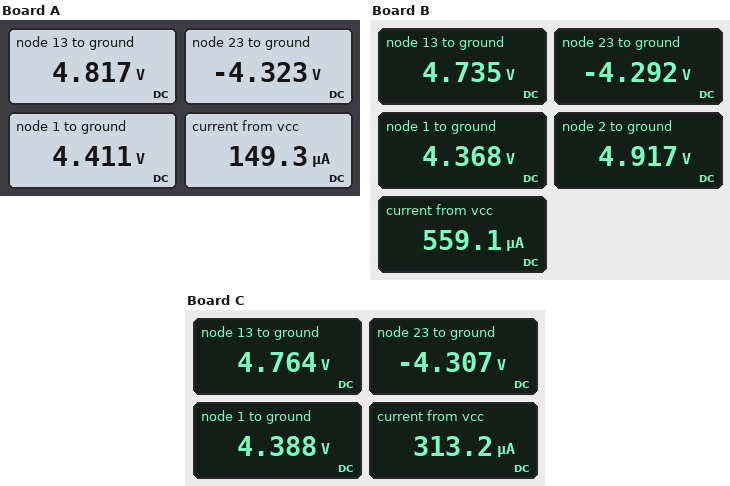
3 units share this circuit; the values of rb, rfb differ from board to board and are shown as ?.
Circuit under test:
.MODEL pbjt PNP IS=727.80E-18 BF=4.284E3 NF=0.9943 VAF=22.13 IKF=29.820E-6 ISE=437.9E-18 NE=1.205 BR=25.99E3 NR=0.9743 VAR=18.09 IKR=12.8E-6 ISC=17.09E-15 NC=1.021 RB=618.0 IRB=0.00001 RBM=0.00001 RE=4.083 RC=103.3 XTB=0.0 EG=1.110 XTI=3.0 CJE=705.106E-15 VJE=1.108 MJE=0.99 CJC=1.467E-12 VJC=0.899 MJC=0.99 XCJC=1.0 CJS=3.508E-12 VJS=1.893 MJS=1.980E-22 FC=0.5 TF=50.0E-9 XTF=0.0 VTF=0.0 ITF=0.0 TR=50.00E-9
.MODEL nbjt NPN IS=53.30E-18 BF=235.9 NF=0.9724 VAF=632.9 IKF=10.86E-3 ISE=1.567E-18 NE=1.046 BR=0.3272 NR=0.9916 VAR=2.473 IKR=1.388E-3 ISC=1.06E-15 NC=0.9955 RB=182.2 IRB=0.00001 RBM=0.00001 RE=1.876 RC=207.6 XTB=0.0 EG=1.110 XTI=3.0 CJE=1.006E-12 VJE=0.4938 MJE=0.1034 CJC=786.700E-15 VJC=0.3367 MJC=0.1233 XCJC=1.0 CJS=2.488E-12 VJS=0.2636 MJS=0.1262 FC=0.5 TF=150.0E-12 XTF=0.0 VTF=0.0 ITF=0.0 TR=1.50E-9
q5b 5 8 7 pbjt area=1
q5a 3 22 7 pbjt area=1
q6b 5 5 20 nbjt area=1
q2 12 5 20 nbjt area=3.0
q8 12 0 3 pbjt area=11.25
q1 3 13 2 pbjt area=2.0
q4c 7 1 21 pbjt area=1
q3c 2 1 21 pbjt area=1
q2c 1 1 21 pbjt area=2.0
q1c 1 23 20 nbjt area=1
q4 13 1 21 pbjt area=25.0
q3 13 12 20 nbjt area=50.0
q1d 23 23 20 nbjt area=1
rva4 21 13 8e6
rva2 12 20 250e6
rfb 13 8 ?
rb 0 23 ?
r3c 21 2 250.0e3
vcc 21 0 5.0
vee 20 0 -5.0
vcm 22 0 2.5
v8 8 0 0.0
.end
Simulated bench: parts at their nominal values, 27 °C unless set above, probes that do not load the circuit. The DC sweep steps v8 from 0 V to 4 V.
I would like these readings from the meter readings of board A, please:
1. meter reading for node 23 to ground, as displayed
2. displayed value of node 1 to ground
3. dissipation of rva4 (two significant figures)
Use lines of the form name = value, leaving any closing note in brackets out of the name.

meter reading for node 23 to ground, as displayed = -4.323 V
displayed value of node 1 to ground = 4.411 V
dissipation of rva4 = 4.2 nW
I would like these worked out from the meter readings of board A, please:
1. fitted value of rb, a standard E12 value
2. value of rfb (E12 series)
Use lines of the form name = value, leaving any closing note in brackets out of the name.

fitted value of rb, a standard E12 value = 220 kΩ
value of rfb = 39 kΩ
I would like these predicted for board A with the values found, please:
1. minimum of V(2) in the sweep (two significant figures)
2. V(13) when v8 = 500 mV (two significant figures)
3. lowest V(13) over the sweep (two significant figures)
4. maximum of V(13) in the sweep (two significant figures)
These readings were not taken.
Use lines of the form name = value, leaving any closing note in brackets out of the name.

minimum of V(2) in the sweep = 590 mV
V(13) when v8 = 500 mV = 4.8 V
lowest V(13) over the sweep = -37 mV
maximum of V(13) in the sweep = 4.9 V
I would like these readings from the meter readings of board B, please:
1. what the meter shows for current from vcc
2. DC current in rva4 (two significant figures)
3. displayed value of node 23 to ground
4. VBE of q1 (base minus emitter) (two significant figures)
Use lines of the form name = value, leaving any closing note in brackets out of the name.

what the meter shows for current from vcc = 559.1 µA
DC current in rva4 = 33 nA
displayed value of node 23 to ground = -4.292 V
VBE of q1 (base minus emitter) = -180 mV
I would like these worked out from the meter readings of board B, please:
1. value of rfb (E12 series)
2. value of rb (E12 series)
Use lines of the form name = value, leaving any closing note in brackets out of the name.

value of rfb = 10 kΩ
value of rb = 68 kΩ
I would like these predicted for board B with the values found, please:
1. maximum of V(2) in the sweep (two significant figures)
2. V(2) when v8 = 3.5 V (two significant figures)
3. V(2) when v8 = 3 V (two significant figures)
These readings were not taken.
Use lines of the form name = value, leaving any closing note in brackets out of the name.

maximum of V(2) in the sweep = 4.9 V
V(2) when v8 = 3.5 V = 630 mV
V(2) when v8 = 3 V = 630 mV
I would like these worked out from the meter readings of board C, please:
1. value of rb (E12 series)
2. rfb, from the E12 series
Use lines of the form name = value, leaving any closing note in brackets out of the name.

value of rb = 120 kΩ
rfb, from the E12 series = 18 kΩ
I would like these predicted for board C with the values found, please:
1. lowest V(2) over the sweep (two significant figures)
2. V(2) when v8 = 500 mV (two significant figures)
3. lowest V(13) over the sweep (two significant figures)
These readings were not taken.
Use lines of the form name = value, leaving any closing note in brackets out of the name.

lowest V(2) over the sweep = 610 mV
V(2) when v8 = 500 mV = 4.9 V
lowest V(13) over the sweep = -30 mV
